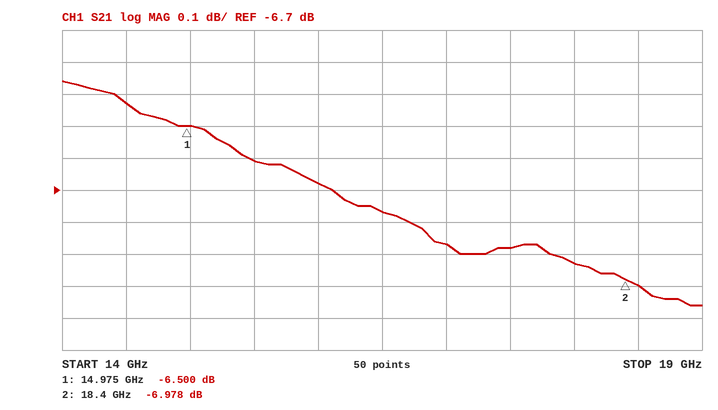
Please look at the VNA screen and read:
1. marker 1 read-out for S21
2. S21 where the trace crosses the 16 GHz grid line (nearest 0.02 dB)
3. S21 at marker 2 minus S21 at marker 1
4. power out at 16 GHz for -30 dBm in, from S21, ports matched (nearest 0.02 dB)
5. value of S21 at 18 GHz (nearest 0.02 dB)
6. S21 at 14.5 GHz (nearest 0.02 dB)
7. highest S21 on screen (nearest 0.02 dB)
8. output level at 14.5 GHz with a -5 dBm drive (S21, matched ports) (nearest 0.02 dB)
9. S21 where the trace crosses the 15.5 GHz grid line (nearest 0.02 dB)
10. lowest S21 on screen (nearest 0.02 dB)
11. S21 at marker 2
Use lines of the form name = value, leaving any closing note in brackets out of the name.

marker 1 read-out for S21 = -6.500 dB
S21 where the trace crosses the 16 GHz grid line = -6.68 dB
S21 at marker 2 minus S21 at marker 1 = -0.478 dB
power out at 16 GHz for -30 dBm in, from S21, ports matched = -36.68 dBm
value of S21 at 18 GHz = -6.92 dB
S21 at 14.5 GHz = -6.42 dB
highest S21 on screen = -6.36 dB
output level at 14.5 GHz with a -5 dBm drive (S21, matched ports) = -11.42 dBm
S21 where the trace crosses the 15.5 GHz grid line = -6.60 dB
lowest S21 on screen = -7.06 dB
S21 at marker 2 = -6.978 dB
